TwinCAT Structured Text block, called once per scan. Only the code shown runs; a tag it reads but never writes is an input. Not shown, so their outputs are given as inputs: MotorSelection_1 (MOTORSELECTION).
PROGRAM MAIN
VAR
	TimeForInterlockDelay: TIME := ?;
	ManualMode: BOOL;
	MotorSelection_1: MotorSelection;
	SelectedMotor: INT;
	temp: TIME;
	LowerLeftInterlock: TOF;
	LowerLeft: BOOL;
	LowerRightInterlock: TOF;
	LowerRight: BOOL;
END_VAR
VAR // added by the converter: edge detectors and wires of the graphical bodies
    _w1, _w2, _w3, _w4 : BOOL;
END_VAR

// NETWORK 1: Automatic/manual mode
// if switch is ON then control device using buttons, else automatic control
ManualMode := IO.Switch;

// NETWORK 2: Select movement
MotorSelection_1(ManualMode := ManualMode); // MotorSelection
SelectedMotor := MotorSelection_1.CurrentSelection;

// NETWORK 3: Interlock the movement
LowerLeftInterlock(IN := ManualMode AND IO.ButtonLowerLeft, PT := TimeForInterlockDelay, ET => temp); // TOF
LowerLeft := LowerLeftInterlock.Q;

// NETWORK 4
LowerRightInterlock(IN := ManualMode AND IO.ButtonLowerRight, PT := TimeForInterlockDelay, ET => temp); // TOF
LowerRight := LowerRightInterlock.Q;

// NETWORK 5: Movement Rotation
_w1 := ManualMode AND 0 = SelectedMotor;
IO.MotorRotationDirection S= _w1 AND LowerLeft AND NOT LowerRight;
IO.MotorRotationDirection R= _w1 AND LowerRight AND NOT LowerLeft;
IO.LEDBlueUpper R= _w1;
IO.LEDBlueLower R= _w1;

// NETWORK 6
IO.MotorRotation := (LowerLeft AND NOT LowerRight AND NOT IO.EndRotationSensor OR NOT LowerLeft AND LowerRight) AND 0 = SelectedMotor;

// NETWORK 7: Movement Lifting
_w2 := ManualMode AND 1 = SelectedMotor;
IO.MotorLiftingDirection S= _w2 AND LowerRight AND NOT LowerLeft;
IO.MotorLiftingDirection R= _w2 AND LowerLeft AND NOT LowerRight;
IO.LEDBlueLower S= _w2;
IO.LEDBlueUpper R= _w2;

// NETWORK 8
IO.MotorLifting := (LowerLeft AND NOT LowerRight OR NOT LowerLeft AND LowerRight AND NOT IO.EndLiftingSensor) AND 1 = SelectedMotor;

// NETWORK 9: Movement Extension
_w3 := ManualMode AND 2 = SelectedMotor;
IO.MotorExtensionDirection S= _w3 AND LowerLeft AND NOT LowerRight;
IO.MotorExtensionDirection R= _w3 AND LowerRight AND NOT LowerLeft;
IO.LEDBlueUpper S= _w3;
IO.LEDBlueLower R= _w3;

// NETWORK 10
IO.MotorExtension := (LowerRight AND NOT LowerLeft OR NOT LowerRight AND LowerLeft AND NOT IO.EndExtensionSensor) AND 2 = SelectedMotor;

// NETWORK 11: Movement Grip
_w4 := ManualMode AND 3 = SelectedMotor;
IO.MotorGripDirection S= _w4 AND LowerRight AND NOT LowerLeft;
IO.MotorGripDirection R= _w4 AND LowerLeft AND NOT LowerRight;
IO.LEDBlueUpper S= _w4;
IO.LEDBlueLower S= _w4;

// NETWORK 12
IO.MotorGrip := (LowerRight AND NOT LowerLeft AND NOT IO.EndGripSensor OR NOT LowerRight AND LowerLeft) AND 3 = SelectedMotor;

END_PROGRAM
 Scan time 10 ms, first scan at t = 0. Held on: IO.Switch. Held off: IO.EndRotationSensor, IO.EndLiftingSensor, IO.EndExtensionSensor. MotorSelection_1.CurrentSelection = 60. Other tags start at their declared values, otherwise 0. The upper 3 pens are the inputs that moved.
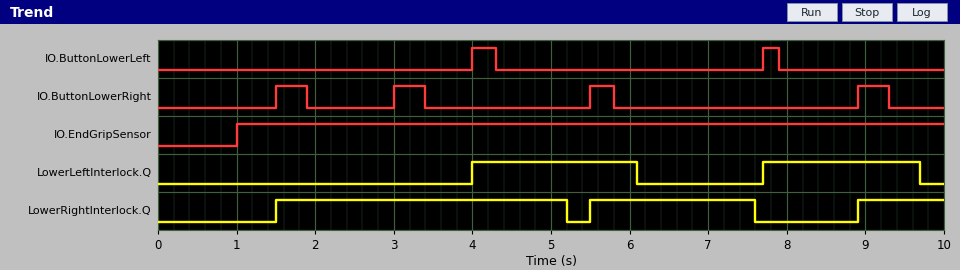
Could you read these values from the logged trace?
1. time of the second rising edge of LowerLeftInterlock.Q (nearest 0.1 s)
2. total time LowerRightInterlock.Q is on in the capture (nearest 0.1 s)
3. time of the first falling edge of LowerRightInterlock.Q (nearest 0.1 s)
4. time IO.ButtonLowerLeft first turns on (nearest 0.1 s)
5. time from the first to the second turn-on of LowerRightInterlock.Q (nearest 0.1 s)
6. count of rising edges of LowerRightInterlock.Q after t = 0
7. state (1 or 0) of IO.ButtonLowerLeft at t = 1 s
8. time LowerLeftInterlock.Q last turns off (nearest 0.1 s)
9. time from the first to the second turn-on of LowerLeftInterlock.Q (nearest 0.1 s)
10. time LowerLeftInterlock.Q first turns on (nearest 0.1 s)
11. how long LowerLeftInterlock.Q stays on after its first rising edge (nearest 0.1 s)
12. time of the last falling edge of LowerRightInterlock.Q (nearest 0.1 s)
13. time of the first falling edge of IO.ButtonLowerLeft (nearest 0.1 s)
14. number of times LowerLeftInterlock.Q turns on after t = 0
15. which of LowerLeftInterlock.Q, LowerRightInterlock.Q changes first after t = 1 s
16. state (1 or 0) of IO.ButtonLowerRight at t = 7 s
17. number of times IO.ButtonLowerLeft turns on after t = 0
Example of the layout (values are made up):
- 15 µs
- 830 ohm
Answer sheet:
- 7.7 s
- 6.9 s
- 5.2 s
- 4.0 s
- 4.0 s
- 3
- 0
- 9.7 s
- 3.7 s
- 4.0 s
- 2.1 s
- 7.6 s
- 4.3 s
- 2
- LowerRightInterlock.Q
- 0
- 2
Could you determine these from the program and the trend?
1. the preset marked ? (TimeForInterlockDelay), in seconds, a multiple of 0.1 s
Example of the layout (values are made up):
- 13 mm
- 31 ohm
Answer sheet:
- 1.8 s
